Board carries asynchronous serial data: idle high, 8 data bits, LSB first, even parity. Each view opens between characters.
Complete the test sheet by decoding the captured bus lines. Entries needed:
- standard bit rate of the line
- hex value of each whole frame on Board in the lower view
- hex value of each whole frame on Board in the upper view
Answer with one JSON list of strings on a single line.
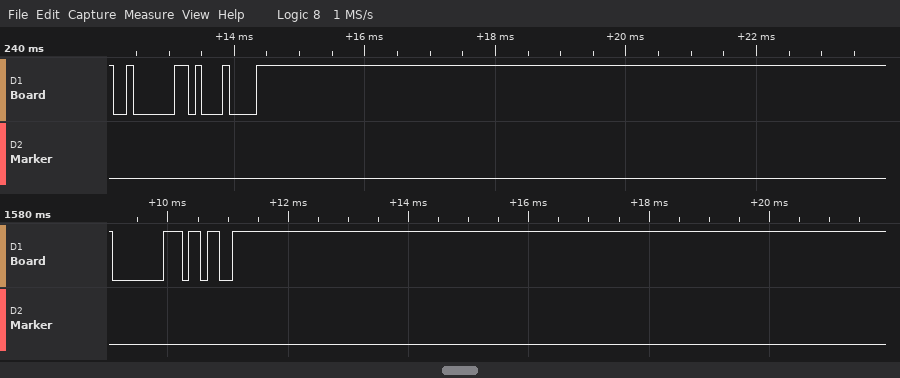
["9600 baud", "80, 9B", "02, 11"]
